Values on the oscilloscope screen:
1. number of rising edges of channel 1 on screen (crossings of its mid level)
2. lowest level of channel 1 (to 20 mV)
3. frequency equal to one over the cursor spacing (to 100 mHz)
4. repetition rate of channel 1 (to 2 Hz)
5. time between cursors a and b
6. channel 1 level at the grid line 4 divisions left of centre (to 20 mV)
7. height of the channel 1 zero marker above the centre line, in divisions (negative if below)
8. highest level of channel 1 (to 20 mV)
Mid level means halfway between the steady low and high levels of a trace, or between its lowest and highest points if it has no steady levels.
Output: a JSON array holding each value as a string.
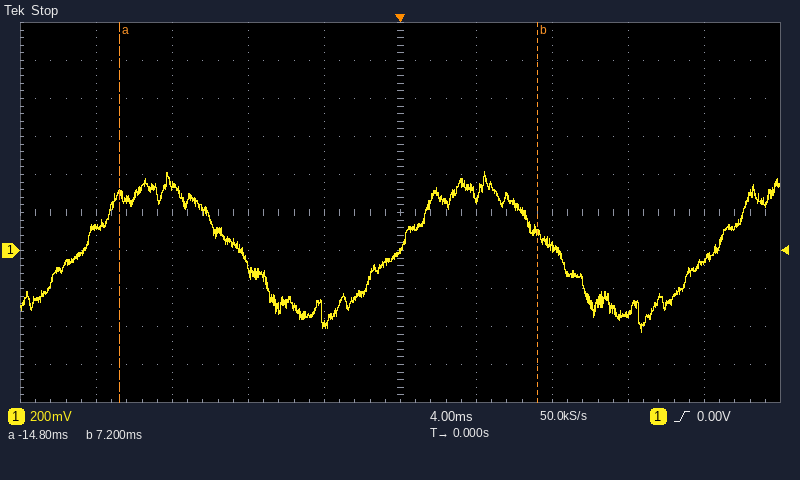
["3", "-440 mV", "45.5 Hz", "60 Hz", "22.0 ms", "120 mV", "-1.0 div", "420 mV"]
